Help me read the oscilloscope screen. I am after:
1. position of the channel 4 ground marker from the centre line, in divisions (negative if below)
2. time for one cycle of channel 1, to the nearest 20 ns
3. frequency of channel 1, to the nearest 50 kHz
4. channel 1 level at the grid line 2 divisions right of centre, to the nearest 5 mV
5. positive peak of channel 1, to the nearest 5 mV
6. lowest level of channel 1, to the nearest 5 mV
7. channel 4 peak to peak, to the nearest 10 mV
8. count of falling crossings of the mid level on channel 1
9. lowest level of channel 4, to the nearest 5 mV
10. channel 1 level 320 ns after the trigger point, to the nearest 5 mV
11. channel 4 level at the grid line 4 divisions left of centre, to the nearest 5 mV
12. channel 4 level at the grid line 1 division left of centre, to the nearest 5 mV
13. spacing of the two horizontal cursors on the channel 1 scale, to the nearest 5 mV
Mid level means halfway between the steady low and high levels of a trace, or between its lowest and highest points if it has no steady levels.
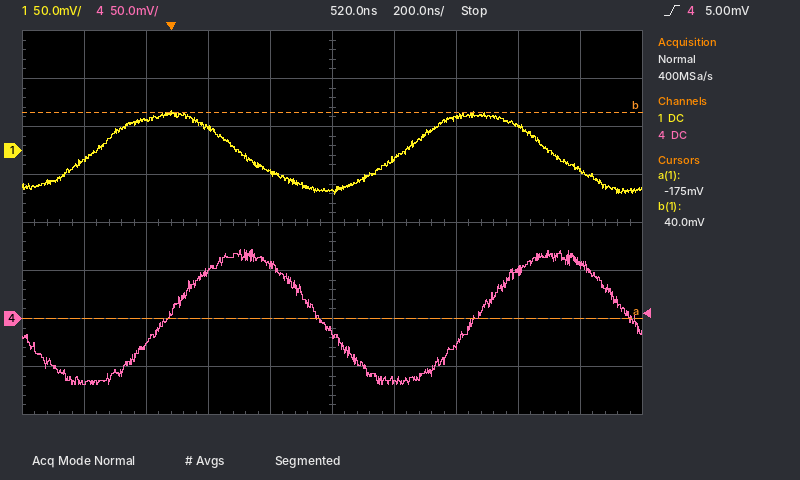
-2.0 div
1.00 µs
1.00 MHz
35 mV
40 mV
-45 mV
140 mV
2
-70 mV
-25 mV
-65 mV
55 mV
215 mV
